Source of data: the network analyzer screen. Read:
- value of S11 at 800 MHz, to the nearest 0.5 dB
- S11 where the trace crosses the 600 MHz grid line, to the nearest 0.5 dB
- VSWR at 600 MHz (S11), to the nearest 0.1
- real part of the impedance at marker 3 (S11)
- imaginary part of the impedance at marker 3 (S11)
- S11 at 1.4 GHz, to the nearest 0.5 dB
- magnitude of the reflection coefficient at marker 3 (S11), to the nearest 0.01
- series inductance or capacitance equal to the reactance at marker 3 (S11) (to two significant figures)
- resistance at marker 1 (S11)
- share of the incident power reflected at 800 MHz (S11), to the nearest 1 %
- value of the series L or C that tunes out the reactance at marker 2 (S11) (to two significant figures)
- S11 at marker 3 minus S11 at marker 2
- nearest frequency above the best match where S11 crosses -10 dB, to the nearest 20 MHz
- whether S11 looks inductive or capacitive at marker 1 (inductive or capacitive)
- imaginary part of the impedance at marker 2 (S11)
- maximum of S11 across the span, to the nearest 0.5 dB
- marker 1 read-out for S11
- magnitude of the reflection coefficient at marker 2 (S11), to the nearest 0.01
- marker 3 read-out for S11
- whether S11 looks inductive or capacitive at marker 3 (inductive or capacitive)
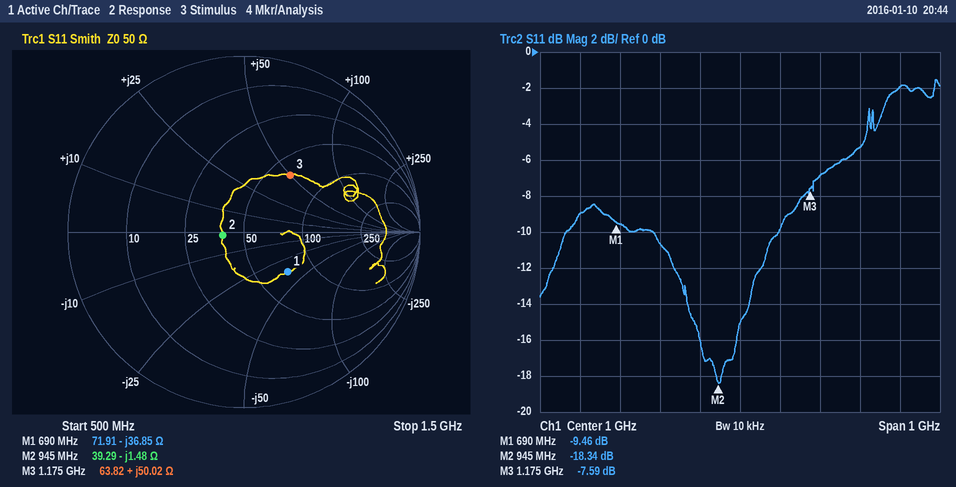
-10.5 dB
-9.0 dB
2.1
63.82 Ω
+50.02 Ω
-2.0 dB
0.42
6.8 nH
71.91 Ω
9 %
250 pH
10.75 dB
1.10 GHz
capacitive
-1.48 Ω
-1.5 dB
-9.46 dB
0.12
-7.59 dB
inductive
